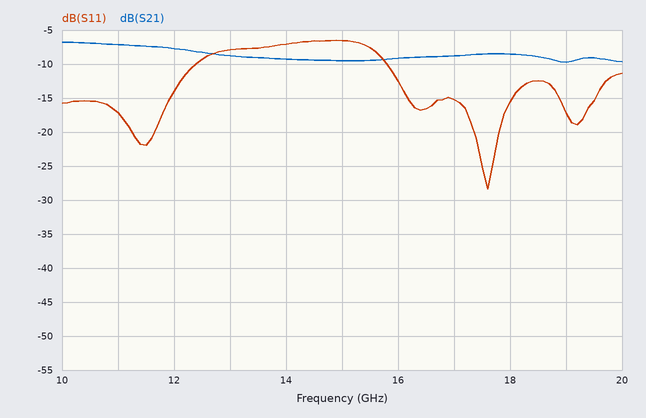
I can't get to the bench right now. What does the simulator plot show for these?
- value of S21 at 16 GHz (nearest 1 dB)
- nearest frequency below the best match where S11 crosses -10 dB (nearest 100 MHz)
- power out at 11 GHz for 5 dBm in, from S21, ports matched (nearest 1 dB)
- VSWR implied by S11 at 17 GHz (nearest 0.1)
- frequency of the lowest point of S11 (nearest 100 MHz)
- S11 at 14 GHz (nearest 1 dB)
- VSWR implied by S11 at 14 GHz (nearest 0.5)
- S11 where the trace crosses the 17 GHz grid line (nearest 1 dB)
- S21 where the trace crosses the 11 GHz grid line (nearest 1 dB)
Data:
-9 dB
15.8 GHz
-2 dBm
1.4
17.6 GHz
-7 dB
2.5
-15 dB
-7 dB
